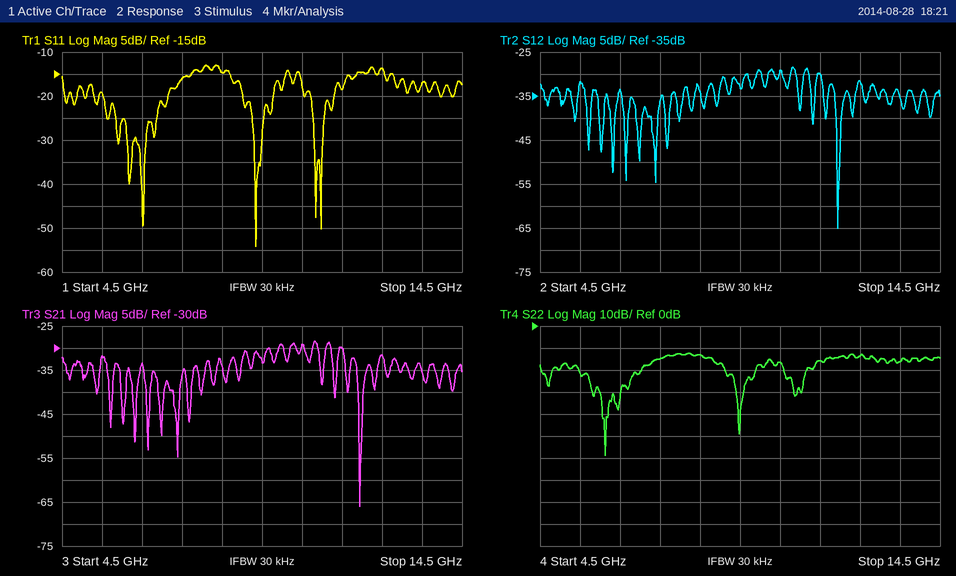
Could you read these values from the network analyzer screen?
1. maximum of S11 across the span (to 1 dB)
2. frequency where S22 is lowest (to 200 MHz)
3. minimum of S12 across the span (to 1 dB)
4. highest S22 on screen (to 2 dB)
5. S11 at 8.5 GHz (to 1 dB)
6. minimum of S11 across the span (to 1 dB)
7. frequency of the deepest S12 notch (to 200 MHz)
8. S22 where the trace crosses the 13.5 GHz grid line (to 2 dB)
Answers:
-13 dB
6.2 GHz
-65 dB
-12 dB
-15 dB
-54 dB
12.0 GHz
-16 dB
